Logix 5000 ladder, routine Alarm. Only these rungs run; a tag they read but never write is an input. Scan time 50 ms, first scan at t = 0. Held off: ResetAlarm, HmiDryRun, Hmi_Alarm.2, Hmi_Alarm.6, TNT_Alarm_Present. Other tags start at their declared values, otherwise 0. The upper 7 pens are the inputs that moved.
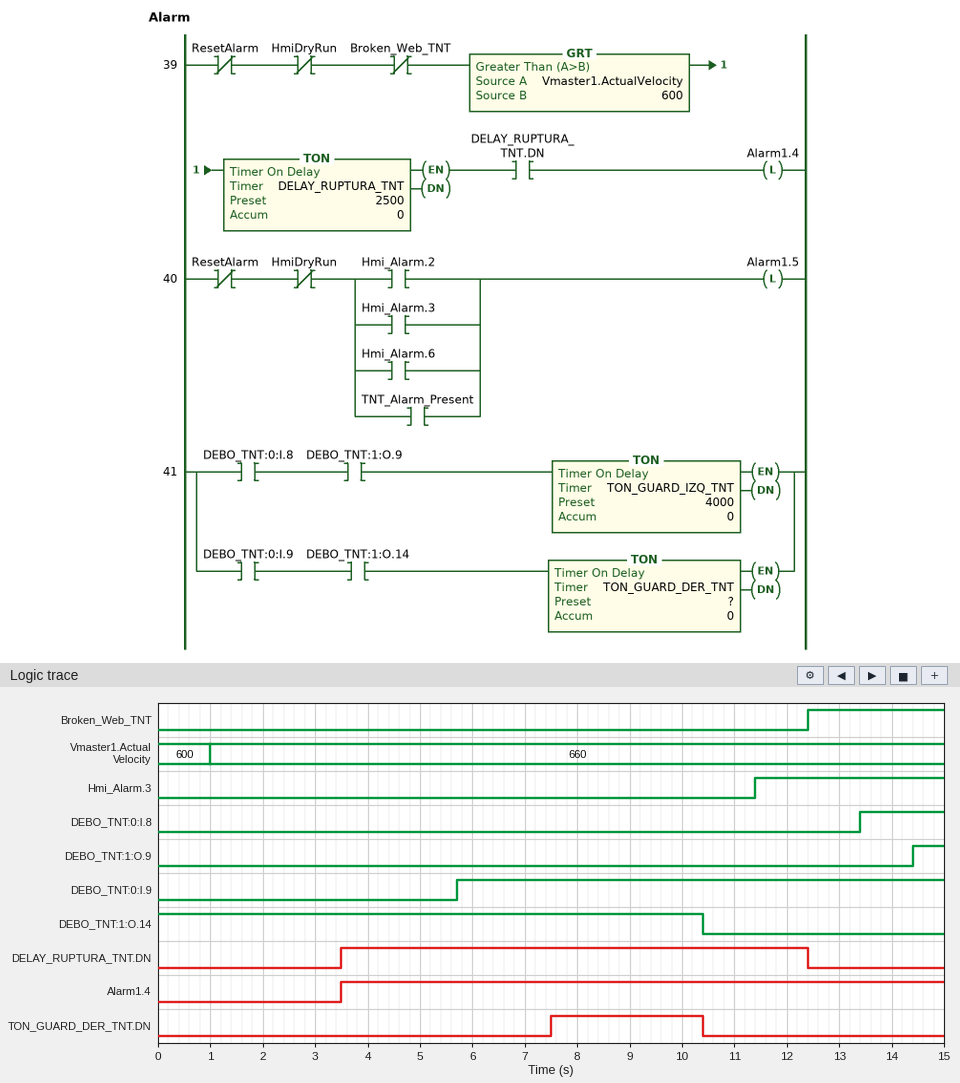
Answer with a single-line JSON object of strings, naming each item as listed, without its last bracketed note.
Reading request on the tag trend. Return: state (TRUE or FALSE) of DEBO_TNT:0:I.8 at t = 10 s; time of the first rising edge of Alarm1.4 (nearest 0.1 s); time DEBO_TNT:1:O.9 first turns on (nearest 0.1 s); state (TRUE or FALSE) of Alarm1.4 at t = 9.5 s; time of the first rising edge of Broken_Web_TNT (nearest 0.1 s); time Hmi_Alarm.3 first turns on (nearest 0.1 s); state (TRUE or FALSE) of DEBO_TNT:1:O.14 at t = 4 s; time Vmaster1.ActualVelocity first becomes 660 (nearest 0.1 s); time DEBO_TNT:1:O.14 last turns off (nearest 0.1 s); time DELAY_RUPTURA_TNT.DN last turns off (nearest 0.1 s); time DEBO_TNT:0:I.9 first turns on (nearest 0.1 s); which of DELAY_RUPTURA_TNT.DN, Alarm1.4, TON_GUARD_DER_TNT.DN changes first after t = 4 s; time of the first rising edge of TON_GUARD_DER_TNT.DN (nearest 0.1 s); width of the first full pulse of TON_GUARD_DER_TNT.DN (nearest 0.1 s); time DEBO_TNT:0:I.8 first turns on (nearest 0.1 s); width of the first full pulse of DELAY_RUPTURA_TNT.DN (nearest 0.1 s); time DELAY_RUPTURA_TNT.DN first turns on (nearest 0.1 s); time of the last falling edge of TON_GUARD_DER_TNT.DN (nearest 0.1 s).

{"state (TRUE or FALSE) of DEBO_TNT:0:I.8 at t = 10 s": "FALSE", "time of the first rising edge of Alarm1.4": "3.5 s", "time DEBO_TNT:1:O.9 first turns on": "14.4 s", "state (TRUE or FALSE) of Alarm1.4 at t = 9.5 s": "TRUE", "time of the first rising edge of Broken_Web_TNT": "12.4 s", "time Hmi_Alarm.3 first turns on": "11.4 s", "state (TRUE or FALSE) of DEBO_TNT:1:O.14 at t = 4 s": "TRUE", "time Vmaster1.ActualVelocity first becomes 660": "1.0 s", "time DEBO_TNT:1:O.14 last turns off": "10.4 s", "time DELAY_RUPTURA_TNT.DN last turns off": "12.4 s", "time DEBO_TNT:0:I.9 first turns on": "5.7 s", "which of DELAY_RUPTURA_TNT.DN, Alarm1.4, TON_GUARD_DER_TNT.DN changes first after t = 4 s": "TON_GUARD_DER_TNT.DN", "time of the first rising edge of TON_GUARD_DER_TNT.DN": "7.5 s", "width of the first full pulse of TON_GUARD_DER_TNT.DN": "2.9 s", "time DEBO_TNT:0:I.8 first turns on": "13.4 s", "width of the first full pulse of DELAY_RUPTURA_TNT.DN": "8.9 s", "time DELAY_RUPTURA_TNT.DN first turns on": "3.5 s", "time of the last falling edge of TON_GUARD_DER_TNT.DN": "10.4 s"}
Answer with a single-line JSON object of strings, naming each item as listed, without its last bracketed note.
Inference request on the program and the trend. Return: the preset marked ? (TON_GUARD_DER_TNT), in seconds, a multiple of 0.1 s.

{"the preset marked ? (TON_GUARD_DER_TNT), in seconds, a multiple of 0.1 s": "1.8 s"}
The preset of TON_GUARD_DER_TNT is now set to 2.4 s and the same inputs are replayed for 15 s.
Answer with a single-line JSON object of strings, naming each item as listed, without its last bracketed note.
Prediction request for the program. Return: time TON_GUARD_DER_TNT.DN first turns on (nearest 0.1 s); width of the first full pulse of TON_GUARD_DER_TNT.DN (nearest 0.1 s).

{"time TON_GUARD_DER_TNT.DN first turns on": "8.1 s", "width of the first full pulse of TON_GUARD_DER_TNT.DN": "2.3 s"}
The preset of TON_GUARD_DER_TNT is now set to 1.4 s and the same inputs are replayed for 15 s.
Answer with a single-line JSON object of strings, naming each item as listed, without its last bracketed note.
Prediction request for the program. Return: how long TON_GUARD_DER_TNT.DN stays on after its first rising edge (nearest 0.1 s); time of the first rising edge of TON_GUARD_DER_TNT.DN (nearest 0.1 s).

{"how long TON_GUARD_DER_TNT.DN stays on after its first rising edge": "3.3 s", "time of the first rising edge of TON_GUARD_DER_TNT.DN": "7.1 s"}
